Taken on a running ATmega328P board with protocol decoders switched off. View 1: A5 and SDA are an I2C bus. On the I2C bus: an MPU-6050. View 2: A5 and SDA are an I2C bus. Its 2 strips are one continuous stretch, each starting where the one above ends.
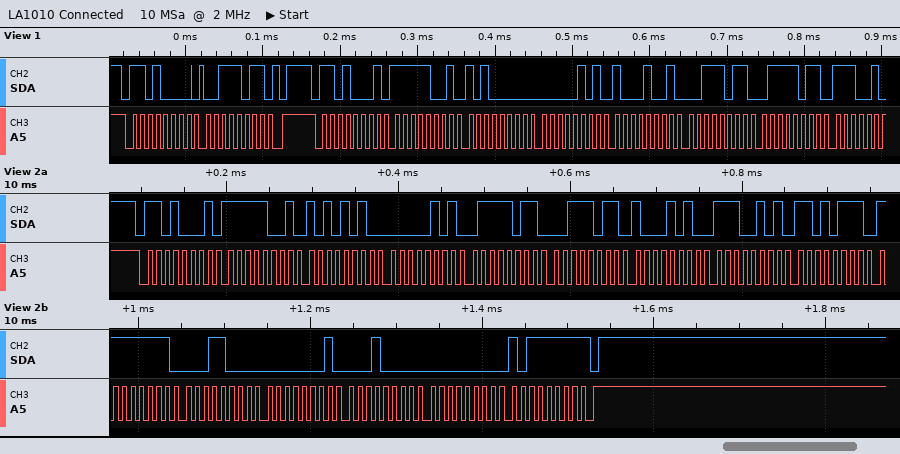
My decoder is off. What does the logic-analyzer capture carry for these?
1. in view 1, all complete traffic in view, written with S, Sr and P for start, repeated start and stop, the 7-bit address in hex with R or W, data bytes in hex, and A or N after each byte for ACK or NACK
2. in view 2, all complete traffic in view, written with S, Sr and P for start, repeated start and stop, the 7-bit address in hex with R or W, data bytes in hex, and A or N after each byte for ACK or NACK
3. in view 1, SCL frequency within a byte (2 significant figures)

S 68W A 3B A P S 68R A F9 A A0 A 05 A 89 A 3B A 7B A
S 68R A F9 A AA A 05 A 7B A 3B A 8A A E5 A D7 A FF A 18 A 01 A 10 A 00 A BF N P
100 kHz
